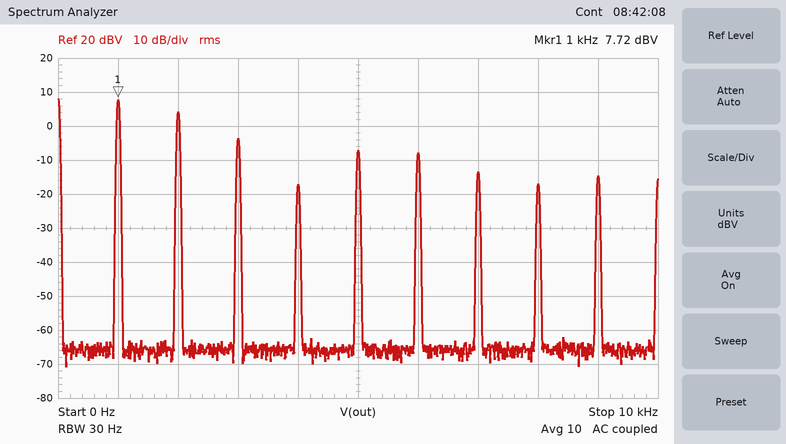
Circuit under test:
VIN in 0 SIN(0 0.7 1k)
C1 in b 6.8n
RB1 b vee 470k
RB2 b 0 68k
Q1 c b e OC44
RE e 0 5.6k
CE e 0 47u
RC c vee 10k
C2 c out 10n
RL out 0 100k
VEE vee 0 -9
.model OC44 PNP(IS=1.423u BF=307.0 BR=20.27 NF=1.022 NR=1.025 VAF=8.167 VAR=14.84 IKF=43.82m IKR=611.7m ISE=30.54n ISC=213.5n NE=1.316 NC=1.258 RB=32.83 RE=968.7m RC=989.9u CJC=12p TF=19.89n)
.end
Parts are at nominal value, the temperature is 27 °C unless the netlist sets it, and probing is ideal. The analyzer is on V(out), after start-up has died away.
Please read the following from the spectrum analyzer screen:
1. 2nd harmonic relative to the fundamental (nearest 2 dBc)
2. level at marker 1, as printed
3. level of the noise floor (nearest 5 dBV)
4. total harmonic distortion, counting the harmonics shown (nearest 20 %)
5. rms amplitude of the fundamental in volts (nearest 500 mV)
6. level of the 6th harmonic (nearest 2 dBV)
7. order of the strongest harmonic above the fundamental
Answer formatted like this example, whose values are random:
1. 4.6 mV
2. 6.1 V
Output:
1. -4 dBc
2. 7.72 dBV
3. -65 dBV
4. 80 %
5. 2.5 V
6. -8 dBV
7. 2
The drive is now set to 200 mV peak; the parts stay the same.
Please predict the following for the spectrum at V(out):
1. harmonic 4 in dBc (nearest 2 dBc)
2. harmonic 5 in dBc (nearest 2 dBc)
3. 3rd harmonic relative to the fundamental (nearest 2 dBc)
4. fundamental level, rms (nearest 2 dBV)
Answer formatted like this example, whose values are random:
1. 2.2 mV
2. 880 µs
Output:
1. -20 dBc
2. -22 dBc
3. -12 dBc
4. 6 dBV
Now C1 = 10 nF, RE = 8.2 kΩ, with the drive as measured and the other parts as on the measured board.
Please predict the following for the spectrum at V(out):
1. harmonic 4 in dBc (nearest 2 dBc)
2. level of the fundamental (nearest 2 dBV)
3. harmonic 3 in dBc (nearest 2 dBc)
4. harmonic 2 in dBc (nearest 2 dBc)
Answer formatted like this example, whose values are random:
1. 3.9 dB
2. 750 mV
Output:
1. -16 dBc
2. 6 dBV
3. -6 dBc
4. -2 dBc
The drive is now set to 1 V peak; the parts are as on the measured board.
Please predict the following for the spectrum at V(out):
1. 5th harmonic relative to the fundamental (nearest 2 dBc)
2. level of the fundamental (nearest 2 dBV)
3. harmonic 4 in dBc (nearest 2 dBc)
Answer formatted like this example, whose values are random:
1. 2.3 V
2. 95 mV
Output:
1. -14 dBc
2. 8 dBV
3. -22 dBc
